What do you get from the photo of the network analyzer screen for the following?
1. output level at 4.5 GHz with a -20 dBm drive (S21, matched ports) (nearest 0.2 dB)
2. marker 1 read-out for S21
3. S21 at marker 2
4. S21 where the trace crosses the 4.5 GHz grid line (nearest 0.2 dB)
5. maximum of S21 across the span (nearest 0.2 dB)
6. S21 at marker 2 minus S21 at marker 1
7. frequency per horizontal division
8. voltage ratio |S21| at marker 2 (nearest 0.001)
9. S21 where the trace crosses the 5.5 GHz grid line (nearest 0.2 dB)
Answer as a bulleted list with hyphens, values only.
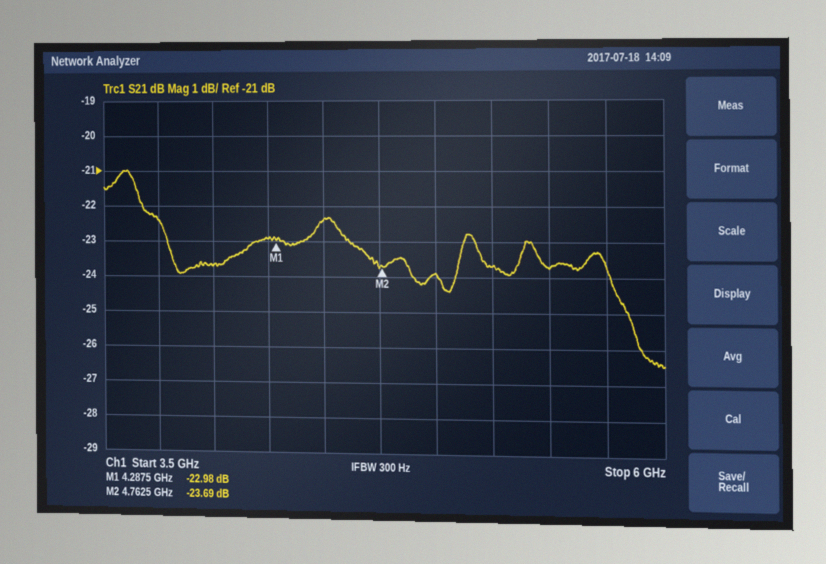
- -42.4 dBm
- -22.98 dB
- -23.69 dB
- -22.4 dB
- -21.0 dB
- -0.71 dB
- 250 MHz
- 0.065
- -23.8 dB
